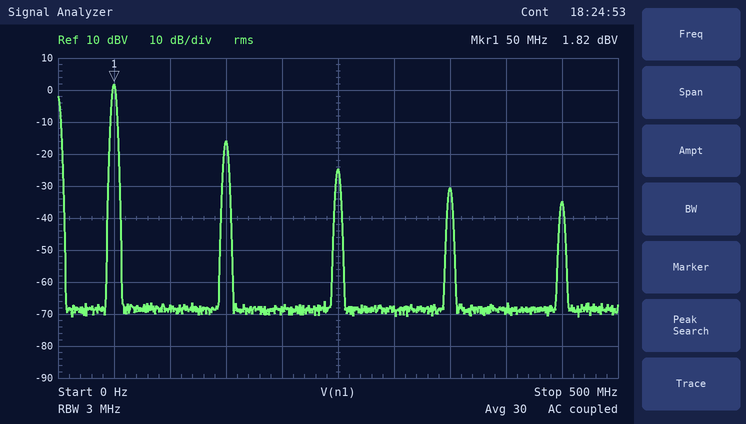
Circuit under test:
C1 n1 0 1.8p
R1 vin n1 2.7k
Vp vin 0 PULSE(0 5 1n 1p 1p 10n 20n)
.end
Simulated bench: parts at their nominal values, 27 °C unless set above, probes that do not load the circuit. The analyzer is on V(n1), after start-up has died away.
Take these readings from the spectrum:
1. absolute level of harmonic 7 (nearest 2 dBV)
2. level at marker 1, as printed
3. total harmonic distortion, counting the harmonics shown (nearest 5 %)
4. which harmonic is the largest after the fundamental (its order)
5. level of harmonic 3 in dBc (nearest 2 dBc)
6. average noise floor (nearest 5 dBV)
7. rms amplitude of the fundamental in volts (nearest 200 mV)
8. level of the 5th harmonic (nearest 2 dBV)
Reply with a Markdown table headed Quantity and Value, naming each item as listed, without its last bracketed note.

| Quantity | Value |
|---|---|
| absolute level of harmonic 7 | -30 dBV |
| level at marker 1, as printed | 1.82 dBV |
| total harmonic distortion, counting the harmonics shown | 15 % |
| which harmonic is the largest after the fundamental | 3 |
| level of harmonic 3 in dBc | -18 dBc |
| average noise floor | -70 dBV |
| rms amplitude of the fundamental in volts | 1.2 V |
| level of the 5th harmonic | -24 dBV |
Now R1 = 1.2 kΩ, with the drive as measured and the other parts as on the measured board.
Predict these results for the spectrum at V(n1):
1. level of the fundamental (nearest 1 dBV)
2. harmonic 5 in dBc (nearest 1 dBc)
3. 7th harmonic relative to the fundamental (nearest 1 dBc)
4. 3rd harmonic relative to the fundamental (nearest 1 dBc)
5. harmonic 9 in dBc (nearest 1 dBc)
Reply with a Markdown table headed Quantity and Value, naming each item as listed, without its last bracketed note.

| Quantity | Value |
|---|---|
| level of the fundamental | 5 dBV |
| harmonic 5 in dBc | -23 dBc |
| 7th harmonic relative to the fundamental | -29 dBc |
| 3rd harmonic relative to the fundamental | -15 dBc |
| harmonic 9 in dBc | -33 dBc |
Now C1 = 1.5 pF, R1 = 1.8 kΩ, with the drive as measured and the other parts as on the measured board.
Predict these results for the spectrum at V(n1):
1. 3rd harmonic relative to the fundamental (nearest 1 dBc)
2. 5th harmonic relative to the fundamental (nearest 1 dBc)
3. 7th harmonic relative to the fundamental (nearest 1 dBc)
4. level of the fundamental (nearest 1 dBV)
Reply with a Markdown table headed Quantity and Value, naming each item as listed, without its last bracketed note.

| Quantity | Value |
|---|---|
| 3rd harmonic relative to the fundamental | -16 dBc |
| 5th harmonic relative to the fundamental | -24 dBc |
| 7th harmonic relative to the fundamental | -30 dBc |
| level of the fundamental | 5 dBV |
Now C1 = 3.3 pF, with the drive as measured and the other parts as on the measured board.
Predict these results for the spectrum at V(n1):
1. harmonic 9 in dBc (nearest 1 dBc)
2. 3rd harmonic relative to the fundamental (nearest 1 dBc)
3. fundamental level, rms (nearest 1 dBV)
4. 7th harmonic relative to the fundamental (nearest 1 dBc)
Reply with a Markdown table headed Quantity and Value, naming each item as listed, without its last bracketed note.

| Quantity | Value |
|---|---|
| harmonic 9 in dBc | -38 dBc |
| 3rd harmonic relative to the fundamental | -19 dBc |
| fundamental level, rms | -2 dBV |
| 7th harmonic relative to the fundamental | -33 dBc |
